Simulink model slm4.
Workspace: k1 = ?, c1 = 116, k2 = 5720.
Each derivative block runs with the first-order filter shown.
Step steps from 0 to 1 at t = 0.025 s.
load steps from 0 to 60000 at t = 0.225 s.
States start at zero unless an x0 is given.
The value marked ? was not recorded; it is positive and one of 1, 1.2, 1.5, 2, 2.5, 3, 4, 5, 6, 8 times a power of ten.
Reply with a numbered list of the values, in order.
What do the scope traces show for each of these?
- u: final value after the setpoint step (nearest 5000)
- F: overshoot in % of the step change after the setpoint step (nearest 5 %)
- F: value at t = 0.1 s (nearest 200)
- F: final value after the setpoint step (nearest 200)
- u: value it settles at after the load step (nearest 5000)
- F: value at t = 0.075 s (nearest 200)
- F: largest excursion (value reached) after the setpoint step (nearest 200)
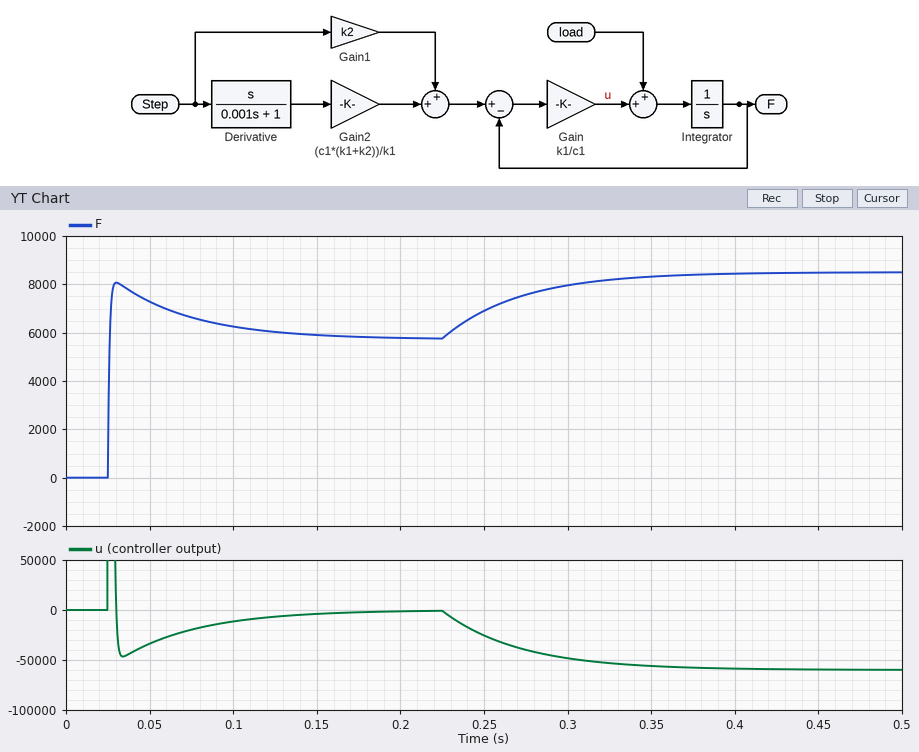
1. 0
2. 40 %
3. 6200
4. 5800
5. -60000
6. 6600
7. 8000
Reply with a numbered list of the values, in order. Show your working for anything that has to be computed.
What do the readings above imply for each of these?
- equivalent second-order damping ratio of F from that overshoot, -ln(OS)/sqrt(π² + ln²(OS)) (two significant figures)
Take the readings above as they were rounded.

1. ln(0.4) = -0.916; 0.916 / sqrt(9.870 + 0.840) = 0.28
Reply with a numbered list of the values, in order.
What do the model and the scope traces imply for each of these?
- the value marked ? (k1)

1. 2500
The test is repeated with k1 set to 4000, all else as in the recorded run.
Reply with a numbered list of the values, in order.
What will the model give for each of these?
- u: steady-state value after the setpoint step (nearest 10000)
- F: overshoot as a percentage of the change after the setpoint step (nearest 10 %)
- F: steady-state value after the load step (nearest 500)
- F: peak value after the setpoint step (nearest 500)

1. 0
2. 60 %
3. 7500
4. 9500
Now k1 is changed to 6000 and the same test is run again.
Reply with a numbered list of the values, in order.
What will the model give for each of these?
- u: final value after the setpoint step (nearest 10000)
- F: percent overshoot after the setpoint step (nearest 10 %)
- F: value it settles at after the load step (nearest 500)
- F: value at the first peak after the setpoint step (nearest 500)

1. 0
2. 90 %
3. 7000
4. 11000
